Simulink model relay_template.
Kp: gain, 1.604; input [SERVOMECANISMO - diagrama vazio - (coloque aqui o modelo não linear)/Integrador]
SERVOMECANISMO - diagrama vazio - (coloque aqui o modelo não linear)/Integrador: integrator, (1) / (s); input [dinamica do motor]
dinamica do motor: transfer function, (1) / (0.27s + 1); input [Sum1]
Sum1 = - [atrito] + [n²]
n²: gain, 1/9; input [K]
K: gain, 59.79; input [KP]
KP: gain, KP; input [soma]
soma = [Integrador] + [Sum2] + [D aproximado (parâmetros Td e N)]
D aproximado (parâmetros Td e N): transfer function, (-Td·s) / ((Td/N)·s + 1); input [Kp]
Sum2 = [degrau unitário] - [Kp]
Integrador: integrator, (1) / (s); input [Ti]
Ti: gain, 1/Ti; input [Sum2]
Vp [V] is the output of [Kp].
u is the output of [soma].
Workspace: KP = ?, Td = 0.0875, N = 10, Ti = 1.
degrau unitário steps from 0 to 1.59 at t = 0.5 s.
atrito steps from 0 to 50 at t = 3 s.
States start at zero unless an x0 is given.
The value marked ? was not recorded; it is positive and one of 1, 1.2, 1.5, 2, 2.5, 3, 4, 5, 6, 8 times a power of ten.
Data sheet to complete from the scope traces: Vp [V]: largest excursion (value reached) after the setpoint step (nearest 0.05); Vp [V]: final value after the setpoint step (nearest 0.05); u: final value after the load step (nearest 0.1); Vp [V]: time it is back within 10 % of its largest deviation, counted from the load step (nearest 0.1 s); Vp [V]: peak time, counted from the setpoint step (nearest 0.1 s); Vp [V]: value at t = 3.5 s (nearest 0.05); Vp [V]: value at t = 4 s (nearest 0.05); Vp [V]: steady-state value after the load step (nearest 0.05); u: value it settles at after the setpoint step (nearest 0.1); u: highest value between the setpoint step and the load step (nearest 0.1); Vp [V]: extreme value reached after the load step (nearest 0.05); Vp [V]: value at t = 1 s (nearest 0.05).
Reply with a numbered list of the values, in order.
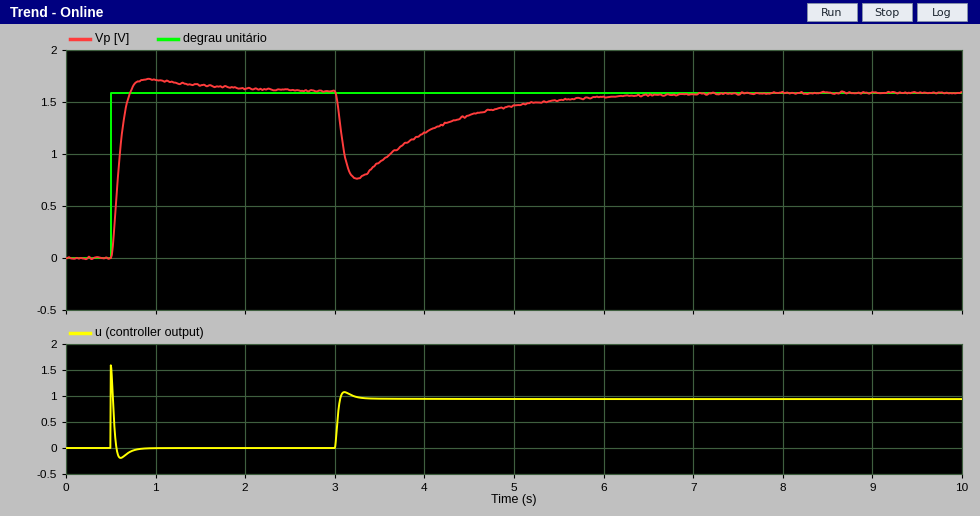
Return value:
1. 1.70
2. 1.60
3. 0.9
4. 2.4 s
5. 0.4 s
6. 0.90
7. 1.20
8. 1.60
9. 0.0
10. 1.6
11. 0.75
12. 1.70
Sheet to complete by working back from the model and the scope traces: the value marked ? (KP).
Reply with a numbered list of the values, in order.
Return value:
1. 8
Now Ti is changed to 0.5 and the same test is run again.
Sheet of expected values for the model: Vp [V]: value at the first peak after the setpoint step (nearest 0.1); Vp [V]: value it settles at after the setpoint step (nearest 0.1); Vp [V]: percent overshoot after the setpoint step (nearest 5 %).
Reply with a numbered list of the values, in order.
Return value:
1. 1.8
2. 1.6
3. 15 %
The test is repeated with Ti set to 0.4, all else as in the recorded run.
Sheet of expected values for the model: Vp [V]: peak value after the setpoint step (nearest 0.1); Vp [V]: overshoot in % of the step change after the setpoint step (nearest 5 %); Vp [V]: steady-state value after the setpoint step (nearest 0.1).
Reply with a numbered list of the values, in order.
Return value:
1. 1.9
2. 15 %
3. 1.6
